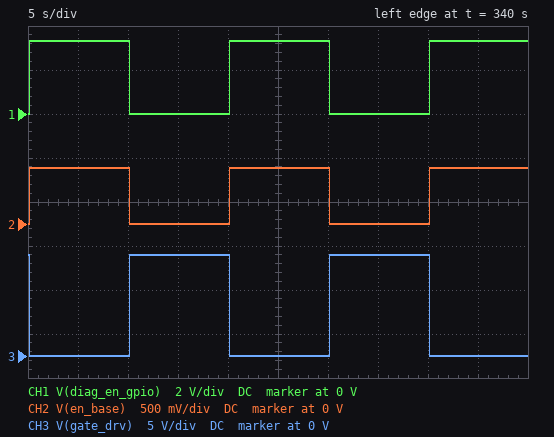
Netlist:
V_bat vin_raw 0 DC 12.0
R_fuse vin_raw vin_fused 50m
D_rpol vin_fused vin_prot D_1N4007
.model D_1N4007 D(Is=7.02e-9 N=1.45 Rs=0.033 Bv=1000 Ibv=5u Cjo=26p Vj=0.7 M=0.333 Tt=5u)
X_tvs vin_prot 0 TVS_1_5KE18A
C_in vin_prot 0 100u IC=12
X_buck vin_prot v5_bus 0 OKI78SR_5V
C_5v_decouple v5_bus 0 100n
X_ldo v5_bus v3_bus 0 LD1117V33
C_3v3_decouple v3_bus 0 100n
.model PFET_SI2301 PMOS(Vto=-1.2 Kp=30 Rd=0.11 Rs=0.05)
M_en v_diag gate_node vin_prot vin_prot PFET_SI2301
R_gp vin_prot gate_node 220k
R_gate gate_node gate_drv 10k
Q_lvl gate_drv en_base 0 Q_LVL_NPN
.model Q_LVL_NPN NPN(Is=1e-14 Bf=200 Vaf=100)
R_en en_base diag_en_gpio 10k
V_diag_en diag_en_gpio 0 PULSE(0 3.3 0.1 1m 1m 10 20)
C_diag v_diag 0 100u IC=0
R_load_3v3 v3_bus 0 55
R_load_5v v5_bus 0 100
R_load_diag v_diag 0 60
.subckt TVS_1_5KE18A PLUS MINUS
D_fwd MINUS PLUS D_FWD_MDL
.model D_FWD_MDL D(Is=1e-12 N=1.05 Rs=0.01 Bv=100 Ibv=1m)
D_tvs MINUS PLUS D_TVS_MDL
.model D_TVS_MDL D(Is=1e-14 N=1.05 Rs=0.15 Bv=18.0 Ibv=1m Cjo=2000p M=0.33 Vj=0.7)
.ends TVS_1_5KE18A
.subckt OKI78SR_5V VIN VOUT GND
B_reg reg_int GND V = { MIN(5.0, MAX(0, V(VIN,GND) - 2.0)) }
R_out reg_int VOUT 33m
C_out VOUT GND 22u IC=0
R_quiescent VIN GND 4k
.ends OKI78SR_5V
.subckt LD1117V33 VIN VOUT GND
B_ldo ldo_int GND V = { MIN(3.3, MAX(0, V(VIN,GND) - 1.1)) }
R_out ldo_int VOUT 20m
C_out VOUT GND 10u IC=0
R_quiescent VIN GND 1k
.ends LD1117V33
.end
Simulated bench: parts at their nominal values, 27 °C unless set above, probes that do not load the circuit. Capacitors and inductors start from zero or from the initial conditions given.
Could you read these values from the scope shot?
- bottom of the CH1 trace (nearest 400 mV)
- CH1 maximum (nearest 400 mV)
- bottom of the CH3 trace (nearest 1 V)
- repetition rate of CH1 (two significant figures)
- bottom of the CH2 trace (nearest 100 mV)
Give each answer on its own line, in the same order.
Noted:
0 V
3.2 V
0 V
50 mHz
0 V
